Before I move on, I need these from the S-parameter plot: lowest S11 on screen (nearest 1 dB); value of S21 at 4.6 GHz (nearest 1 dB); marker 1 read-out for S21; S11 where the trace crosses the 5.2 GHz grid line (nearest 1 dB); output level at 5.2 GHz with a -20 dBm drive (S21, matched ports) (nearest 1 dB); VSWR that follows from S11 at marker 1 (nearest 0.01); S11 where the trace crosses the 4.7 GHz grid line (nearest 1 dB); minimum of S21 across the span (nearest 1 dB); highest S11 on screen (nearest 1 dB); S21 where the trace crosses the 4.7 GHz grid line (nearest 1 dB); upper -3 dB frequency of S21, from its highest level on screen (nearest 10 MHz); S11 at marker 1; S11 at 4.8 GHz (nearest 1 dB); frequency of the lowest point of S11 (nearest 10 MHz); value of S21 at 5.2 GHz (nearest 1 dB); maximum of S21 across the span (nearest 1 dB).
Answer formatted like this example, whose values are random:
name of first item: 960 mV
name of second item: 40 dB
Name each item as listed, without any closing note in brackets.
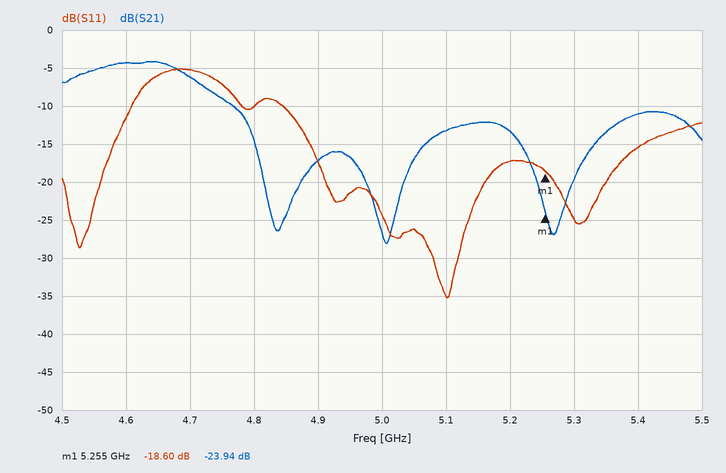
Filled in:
lowest S11 on screen: -35 dB
value of S21 at 4.6 GHz: -4 dB
marker 1 read-out for S21: -23.94 dB
S11 where the trace crosses the 5.2 GHz grid line: -17 dB
output level at 5.2 GHz with a -20 dBm drive (S21, matched ports): -33 dBm
VSWR that follows from S11 at marker 1: 1.27
S11 where the trace crosses the 4.7 GHz grid line: -5 dB
minimum of S21 across the span: -28 dB
highest S11 on screen: -5 dB
S21 where the trace crosses the 4.7 GHz grid line: -6 dB
upper -3 dB frequency of S21, from its highest level on screen: 4.72 GHz
S11 at marker 1: -18.60 dB
S11 at 4.8 GHz: -10 dB
frequency of the lowest point of S11: 5.10 GHz
value of S21 at 5.2 GHz: -13 dB
maximum of S21 across the span: -4 dB
